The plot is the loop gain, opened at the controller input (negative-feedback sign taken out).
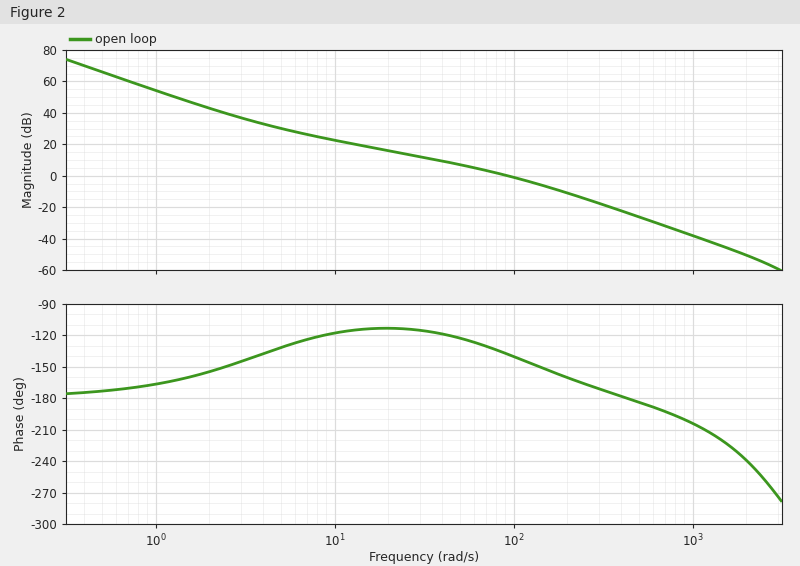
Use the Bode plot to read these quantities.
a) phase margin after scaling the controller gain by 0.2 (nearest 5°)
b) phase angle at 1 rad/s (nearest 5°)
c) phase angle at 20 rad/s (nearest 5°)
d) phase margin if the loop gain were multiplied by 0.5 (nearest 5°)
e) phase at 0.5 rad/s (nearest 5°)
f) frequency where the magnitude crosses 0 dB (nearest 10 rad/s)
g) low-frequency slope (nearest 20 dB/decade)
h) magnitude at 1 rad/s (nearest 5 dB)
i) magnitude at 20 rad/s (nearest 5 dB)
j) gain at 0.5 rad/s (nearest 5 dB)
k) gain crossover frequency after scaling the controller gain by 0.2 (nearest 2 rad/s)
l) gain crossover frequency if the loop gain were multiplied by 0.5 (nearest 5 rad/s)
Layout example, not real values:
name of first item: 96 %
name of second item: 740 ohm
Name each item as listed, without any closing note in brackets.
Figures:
phase margin after scaling the controller gain by 0.2: 65°
phase angle at 1 rad/s: -165°
phase angle at 20 rad/s: -115°
phase margin if the loop gain were multiplied by 0.5: 55°
phase at 0.5 rad/s: -175°
frequency where the magnitude crosses 0 dB: 90 rad/s
low-frequency slope: -40 dB/decade
magnitude at 1 rad/s: 55 dB
magnitude at 20 rad/s: 15 dB
gain at 0.5 rad/s: 65 dB
gain crossover frequency after scaling the controller gain by 0.2: 24 rad/s
gain crossover frequency if the loop gain were multiplied by 0.5: 55 rad/s
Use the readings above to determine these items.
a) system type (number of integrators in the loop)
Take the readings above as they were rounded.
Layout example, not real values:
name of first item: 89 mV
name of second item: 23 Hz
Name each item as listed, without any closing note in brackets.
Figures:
system type: 2
